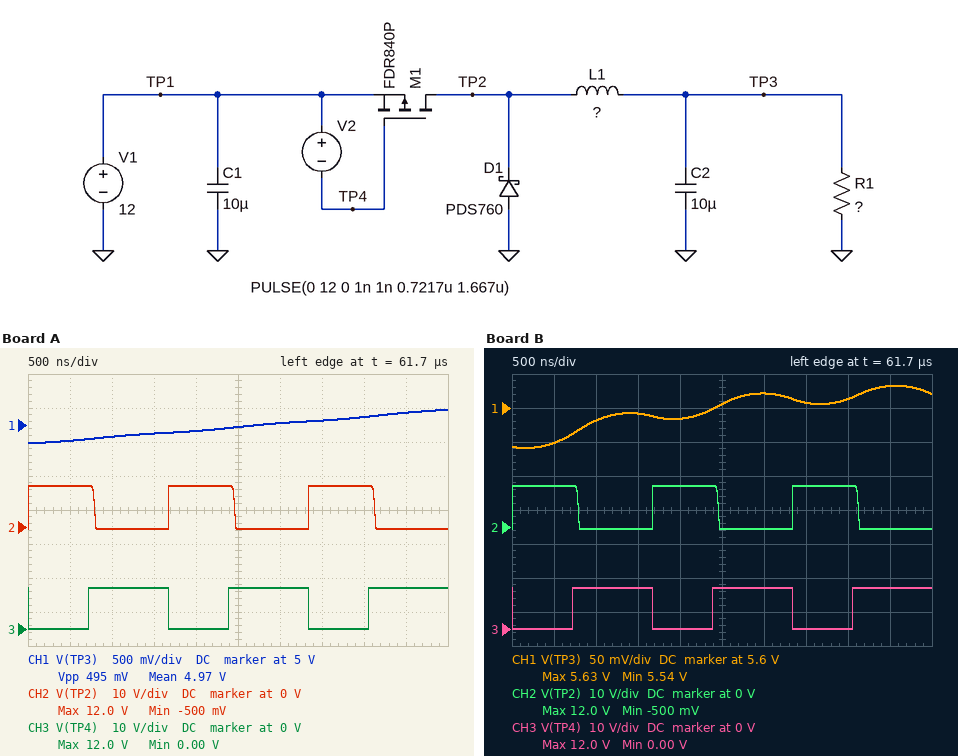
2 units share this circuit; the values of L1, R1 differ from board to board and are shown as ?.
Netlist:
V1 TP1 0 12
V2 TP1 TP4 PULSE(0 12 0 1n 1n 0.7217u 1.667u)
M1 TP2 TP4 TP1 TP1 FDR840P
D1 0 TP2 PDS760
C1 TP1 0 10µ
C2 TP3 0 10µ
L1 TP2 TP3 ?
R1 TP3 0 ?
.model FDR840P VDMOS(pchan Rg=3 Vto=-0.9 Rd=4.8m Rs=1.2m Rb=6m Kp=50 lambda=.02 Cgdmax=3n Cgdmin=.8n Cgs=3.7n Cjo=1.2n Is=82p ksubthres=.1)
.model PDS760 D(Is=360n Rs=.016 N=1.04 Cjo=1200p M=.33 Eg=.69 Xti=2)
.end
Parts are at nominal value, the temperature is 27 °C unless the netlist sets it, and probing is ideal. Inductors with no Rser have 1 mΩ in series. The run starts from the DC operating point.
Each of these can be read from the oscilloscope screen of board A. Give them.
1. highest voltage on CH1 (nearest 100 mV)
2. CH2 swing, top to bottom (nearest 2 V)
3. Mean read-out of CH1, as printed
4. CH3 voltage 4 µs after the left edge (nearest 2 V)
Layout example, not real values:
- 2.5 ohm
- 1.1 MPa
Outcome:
- 5.2 V
- 12 V
- 4.97 V
- 0 V
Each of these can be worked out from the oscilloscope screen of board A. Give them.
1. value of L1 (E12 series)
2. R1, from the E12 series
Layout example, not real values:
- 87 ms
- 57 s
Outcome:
- 6.8 µH
- 2.7 Ω
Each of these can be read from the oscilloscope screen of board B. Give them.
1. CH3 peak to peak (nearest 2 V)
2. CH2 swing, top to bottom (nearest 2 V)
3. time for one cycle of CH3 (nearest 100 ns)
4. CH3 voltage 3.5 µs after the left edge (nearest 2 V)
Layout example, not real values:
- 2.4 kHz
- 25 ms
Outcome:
- 12 V
- 12 V
- 1.7 µs
- 0 V
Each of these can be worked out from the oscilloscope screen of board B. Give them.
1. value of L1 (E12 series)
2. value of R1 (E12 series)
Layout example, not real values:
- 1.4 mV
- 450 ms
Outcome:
- 4.7 µH
- 1.2 Ω
